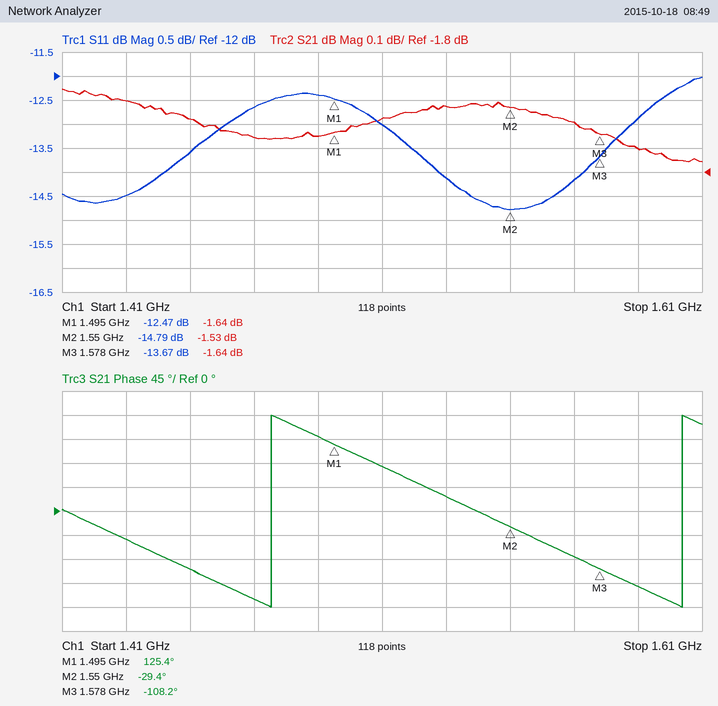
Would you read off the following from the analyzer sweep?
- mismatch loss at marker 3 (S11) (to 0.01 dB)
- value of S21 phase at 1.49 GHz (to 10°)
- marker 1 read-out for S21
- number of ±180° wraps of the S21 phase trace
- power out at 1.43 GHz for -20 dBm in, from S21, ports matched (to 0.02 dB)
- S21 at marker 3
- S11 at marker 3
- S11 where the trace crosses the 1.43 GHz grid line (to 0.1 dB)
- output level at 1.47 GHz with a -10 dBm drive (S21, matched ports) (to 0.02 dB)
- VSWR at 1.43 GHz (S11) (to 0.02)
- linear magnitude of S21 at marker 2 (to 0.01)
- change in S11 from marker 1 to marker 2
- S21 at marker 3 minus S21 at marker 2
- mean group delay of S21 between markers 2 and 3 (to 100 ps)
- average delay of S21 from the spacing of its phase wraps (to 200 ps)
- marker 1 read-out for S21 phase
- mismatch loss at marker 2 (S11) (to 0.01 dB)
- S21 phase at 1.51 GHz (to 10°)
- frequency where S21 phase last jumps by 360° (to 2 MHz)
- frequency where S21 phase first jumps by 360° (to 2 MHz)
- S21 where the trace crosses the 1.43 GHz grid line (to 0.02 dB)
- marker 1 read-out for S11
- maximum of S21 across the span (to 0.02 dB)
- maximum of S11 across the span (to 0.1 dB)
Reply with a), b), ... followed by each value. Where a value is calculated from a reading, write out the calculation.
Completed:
a) −10 log10(1 − 10^(-13.67/10)) ≈ 0.19 dB
b) 140°
c) -1.64 dB
d) 2
e) -20 dBm + (-1.50 dB) = -21.50 dBm
f) -1.64 dB
g) -13.67 dB
h) -14.5 dB
i) -10 dBm + (-1.66 dB) = -11.66 dBm
j) |Γ| = 10^(-14.5/20) = 0.1884; VSWR = (1 + 0.1884)/(1 − 0.1884) ≈ 1.46
k) 10^(-1.53/20) ≈ 0.84
l) -14.79 − (-12.47) = -2.32 dB
m) -1.64 − (-1.53) = -0.11 dB
n) −(-108.2° − (-29.4°))/(360° × 28 MHz) ≈ 7.8 ns
o) 1 cycle / (1.604 GHz − 1.476 GHz) ≈ 7.8 ns
p) 125.4°
q) −10 log10(1 − 10^(-14.79/10)) ≈ 0.15 dB
r) 80°
s) 1.604 GHz
t) 1.476 GHz
u) -1.50 dB
v) -12.47 dB
w) -1.46 dB
x) -12.0 dB
